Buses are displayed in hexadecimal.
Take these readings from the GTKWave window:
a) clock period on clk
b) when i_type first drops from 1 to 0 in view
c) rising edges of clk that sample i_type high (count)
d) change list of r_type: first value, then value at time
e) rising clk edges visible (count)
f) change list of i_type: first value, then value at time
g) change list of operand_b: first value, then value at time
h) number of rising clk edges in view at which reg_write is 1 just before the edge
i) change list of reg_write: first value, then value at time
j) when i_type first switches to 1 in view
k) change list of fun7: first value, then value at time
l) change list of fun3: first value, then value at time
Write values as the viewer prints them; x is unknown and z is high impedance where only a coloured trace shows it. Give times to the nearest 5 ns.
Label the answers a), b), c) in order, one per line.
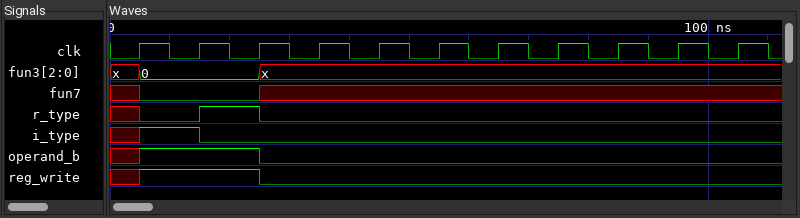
a) 10 ns
b) 15 ns
c) 1
d) x, 0 at 5 ns, 1 at 15 ns, 0 at 25 ns
e) 11
f) x, 1 at 5 ns, 0 at 15 ns
g) x, 1 at 5 ns, 0 at 25 ns
h) 2
i) x, 1 at 5 ns, 0 at 25 ns
j) 5 ns
k) x, 0 at 5 ns, x at 25 ns
l) x, 0 at 5 ns, x at 25 ns
